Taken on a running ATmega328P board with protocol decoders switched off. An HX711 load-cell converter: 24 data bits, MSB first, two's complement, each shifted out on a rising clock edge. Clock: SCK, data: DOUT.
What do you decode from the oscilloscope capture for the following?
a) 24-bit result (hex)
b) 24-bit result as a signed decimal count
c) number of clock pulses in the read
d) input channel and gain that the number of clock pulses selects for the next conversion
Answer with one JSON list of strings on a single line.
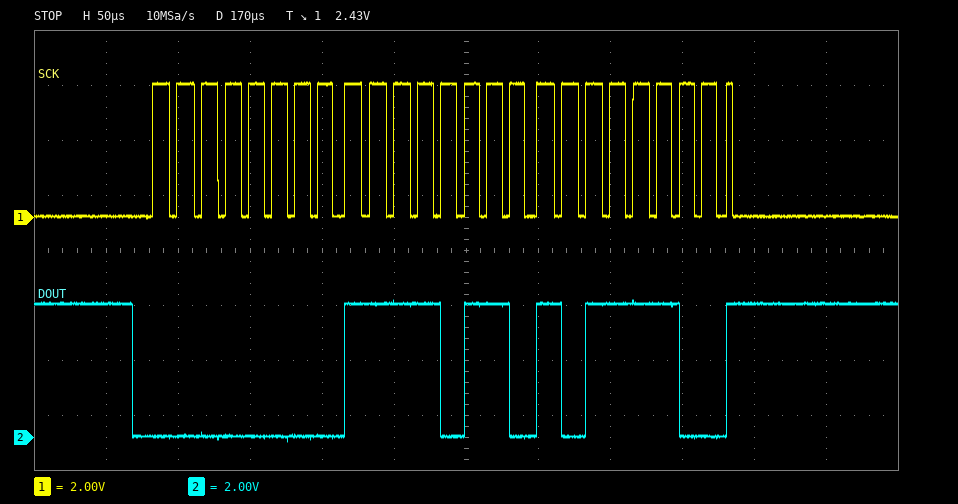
["0x00F6BC", "63164", "25", "channel A, gain 128"]
